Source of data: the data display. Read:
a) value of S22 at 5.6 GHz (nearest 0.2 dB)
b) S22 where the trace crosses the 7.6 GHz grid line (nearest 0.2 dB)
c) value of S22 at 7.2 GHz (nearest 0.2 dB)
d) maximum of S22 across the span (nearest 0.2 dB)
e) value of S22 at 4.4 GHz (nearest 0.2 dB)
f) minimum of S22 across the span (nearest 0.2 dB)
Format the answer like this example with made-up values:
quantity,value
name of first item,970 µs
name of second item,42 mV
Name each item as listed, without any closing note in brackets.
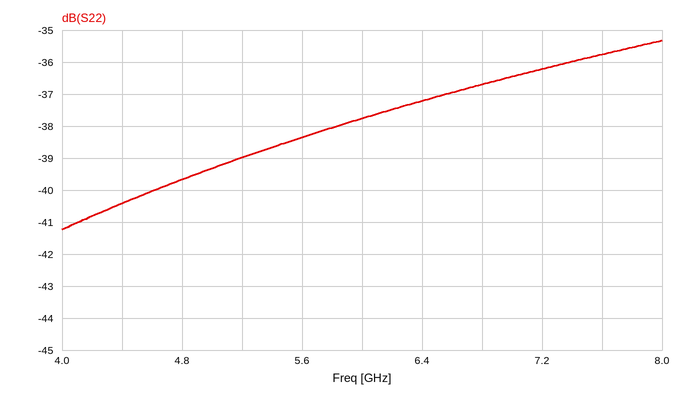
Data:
quantity,value
value of S22 at 5.6 GHz,-38.4 dB
S22 where the trace crosses the 7.6 GHz grid line,-35.8 dB
value of S22 at 7.2 GHz,-36.2 dB
maximum of S22 across the span,-35.4 dB
value of S22 at 4.4 GHz,-40.4 dB
minimum of S22 across the span,-41.2 dB
